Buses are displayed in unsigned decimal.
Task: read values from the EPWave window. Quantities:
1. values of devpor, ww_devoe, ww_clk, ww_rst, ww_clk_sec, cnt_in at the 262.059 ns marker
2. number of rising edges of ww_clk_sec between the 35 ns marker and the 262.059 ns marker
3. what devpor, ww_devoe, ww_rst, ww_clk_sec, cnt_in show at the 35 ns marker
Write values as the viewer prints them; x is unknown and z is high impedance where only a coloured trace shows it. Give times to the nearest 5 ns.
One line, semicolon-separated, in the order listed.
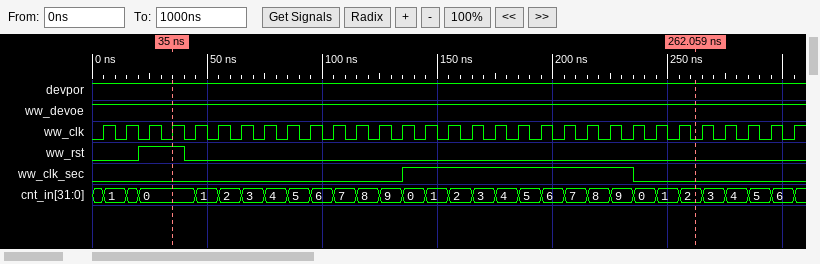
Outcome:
devpor=1, ww_devoe=1, ww_clk=0, ww_rst=0, ww_clk_sec=0, cnt_in=2; 1; devpor=1, ww_devoe=1, ww_rst=1, ww_clk_sec=0, cnt_in=0
